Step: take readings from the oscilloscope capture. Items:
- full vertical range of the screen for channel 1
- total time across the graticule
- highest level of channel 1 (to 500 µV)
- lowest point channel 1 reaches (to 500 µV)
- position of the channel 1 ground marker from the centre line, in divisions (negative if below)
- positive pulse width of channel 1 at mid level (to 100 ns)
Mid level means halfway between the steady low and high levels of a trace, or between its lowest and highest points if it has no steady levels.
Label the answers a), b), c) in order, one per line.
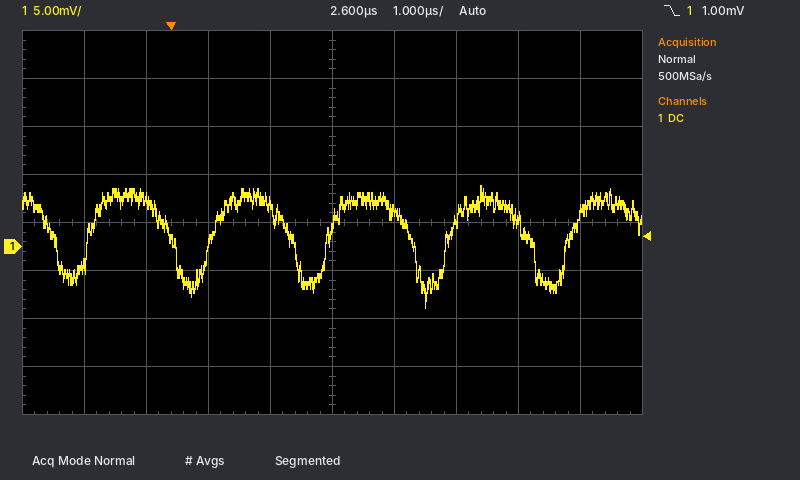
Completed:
a) 40 mV
b) 10 µs
c) 6.5 mV
d) -6.5 mV
e) -0.5 div
f) 1.4 µs
